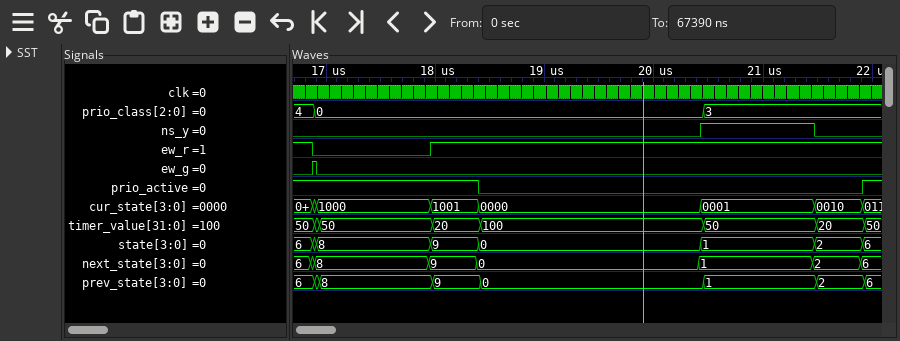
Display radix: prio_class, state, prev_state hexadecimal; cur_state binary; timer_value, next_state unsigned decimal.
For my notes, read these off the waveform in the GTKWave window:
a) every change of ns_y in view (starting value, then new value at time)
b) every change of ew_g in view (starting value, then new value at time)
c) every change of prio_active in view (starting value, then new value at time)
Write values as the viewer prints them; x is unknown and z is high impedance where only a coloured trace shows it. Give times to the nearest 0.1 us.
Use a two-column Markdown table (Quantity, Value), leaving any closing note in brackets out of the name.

| Quantity | Value |
|---|---|
| every change of ns_y in view | 0, 1 at 20.4 us, 0 at 21.5 us |
| every change of ew_g in view | 0, 1 at 16.9 us, 0 at 16.9 us |
| every change of prio_active in view | 1, 0 at 18.4 us, 1 at 21.9 us |
